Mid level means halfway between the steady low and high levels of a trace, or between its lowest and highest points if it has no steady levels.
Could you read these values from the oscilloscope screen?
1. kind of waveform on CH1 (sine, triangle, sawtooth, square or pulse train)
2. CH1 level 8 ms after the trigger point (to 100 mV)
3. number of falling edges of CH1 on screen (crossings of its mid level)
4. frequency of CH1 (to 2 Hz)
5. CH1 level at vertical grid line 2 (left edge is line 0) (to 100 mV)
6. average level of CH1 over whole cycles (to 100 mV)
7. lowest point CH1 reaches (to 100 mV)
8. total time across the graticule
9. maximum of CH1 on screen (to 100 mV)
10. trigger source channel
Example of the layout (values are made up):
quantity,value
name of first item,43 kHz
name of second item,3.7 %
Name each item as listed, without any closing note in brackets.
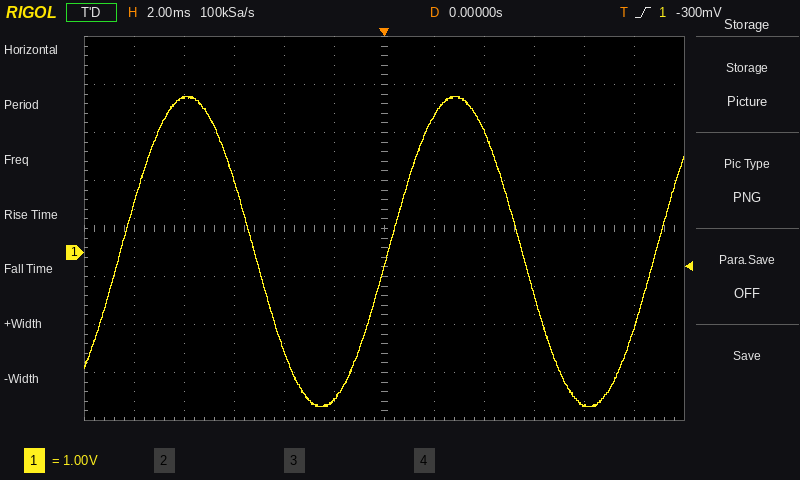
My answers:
quantity,value
kind of waveform on CH1,sine
CH1 level 8 ms after the trigger point,-3.2 V
number of falling edges of CH1 on screen,2
frequency of CH1,94 Hz
CH1 level at vertical grid line 2 (left edge is line 0),3.2 V
average level of CH1 over whole cycles,0.0 V
lowest point CH1 reaches,-3.2 V
total time across the graticule,24 ms
maximum of CH1 on screen,3.2 V
trigger source channel,CH1
